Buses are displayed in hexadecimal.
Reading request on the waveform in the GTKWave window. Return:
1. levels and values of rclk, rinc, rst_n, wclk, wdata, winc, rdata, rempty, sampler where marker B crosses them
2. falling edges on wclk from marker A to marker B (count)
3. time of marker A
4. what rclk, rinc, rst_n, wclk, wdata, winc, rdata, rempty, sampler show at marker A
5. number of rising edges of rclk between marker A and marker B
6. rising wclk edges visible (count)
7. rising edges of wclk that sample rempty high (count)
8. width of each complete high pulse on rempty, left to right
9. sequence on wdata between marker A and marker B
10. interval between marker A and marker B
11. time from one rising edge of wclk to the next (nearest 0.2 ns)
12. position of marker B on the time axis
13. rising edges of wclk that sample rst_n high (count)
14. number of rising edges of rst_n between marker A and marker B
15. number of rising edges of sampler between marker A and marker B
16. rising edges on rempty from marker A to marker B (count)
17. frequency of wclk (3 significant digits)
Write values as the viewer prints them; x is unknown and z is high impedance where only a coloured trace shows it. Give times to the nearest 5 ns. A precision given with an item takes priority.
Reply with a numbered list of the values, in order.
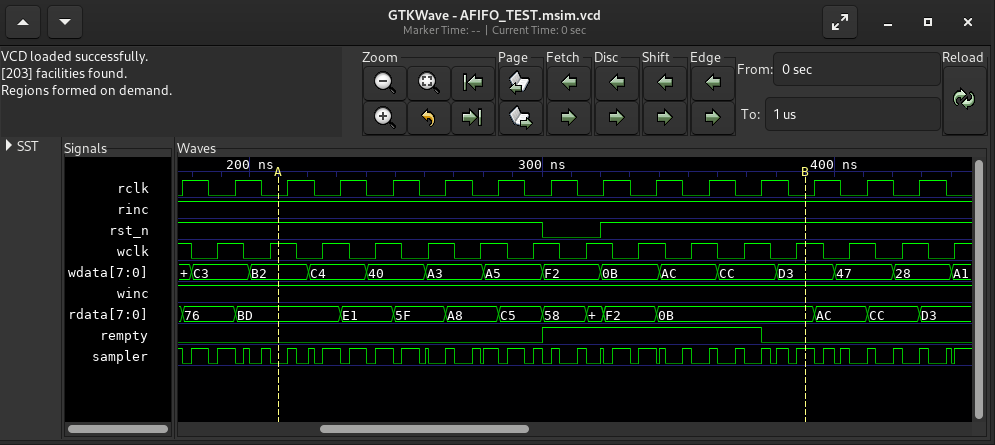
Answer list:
1. rclk=0, rinc=1, rst_n=1, wclk=1, wdata=D3, winc=1, rdata=0B, rempty=0, sampler=1
2. 10
3. 210 ns
4. rclk=0, rinc=1, rst_n=1, wclk=1, wdata=B2, winc=1, rdata=BD, rempty=0, sampler=0
5. 10
6. 15
7. 4
8. 75 ns
9. B2, C4, 40, A3, A5, F2, 0B, AC, CC, D3
10. 180 ns
11. 18 ns
12. 390 ns
13. 14
14. 1
15. 24
16. 1
17. 55.6 MHz
